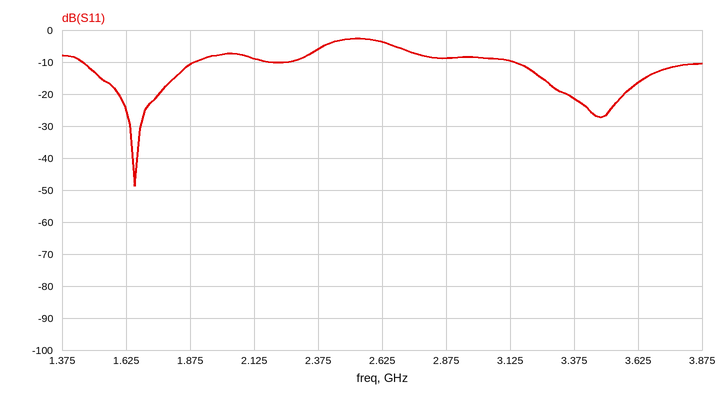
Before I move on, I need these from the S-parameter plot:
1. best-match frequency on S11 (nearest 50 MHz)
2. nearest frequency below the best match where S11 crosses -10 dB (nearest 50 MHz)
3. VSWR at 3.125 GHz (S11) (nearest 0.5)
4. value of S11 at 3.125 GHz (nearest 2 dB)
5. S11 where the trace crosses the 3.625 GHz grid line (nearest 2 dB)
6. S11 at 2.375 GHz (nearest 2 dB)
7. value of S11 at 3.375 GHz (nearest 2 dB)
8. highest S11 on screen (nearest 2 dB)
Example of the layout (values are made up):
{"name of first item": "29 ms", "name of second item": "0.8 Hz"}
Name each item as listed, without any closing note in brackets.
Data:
{"best-match frequency on S11": "1.65 GHz", "nearest frequency below the best match where S11 crosses -10 dB": "1.45 GHz", "VSWR at 3.125 GHz (S11)": "2.0", "value of S11 at 3.125 GHz": "-10 dB", "S11 where the trace crosses the 3.625 GHz grid line": "-16 dB", "S11 at 2.375 GHz": "-6 dB", "value of S11 at 3.375 GHz": "-22 dB", "highest S11 on screen": "-2 dB"}
